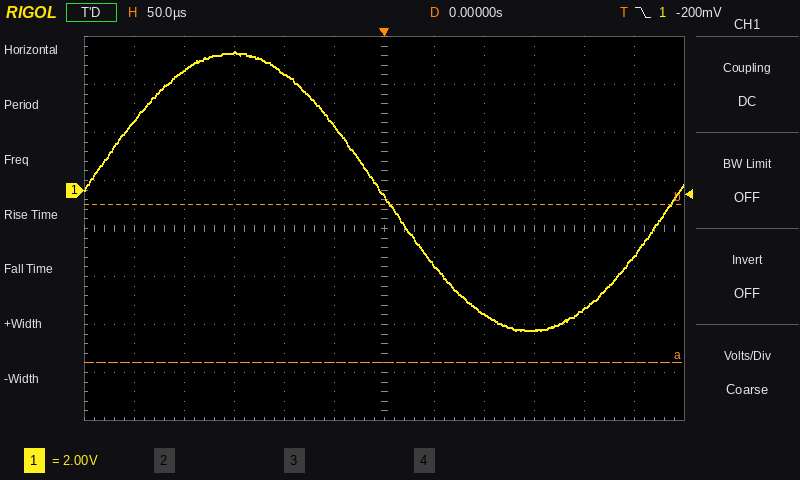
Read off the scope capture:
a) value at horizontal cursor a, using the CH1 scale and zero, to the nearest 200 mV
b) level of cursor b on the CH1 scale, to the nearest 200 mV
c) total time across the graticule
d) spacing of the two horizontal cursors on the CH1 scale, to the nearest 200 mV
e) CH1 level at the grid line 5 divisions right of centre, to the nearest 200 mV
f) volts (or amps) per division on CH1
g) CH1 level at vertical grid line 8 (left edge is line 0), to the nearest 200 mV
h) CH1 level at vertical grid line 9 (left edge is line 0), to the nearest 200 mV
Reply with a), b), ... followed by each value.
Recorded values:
a) -7.2 V
b) -600 mV
c) 600 µs
d) 6.6 V
e) -2.8 V
f) 2 V
g) -5.2 V
h) -5.8 V
